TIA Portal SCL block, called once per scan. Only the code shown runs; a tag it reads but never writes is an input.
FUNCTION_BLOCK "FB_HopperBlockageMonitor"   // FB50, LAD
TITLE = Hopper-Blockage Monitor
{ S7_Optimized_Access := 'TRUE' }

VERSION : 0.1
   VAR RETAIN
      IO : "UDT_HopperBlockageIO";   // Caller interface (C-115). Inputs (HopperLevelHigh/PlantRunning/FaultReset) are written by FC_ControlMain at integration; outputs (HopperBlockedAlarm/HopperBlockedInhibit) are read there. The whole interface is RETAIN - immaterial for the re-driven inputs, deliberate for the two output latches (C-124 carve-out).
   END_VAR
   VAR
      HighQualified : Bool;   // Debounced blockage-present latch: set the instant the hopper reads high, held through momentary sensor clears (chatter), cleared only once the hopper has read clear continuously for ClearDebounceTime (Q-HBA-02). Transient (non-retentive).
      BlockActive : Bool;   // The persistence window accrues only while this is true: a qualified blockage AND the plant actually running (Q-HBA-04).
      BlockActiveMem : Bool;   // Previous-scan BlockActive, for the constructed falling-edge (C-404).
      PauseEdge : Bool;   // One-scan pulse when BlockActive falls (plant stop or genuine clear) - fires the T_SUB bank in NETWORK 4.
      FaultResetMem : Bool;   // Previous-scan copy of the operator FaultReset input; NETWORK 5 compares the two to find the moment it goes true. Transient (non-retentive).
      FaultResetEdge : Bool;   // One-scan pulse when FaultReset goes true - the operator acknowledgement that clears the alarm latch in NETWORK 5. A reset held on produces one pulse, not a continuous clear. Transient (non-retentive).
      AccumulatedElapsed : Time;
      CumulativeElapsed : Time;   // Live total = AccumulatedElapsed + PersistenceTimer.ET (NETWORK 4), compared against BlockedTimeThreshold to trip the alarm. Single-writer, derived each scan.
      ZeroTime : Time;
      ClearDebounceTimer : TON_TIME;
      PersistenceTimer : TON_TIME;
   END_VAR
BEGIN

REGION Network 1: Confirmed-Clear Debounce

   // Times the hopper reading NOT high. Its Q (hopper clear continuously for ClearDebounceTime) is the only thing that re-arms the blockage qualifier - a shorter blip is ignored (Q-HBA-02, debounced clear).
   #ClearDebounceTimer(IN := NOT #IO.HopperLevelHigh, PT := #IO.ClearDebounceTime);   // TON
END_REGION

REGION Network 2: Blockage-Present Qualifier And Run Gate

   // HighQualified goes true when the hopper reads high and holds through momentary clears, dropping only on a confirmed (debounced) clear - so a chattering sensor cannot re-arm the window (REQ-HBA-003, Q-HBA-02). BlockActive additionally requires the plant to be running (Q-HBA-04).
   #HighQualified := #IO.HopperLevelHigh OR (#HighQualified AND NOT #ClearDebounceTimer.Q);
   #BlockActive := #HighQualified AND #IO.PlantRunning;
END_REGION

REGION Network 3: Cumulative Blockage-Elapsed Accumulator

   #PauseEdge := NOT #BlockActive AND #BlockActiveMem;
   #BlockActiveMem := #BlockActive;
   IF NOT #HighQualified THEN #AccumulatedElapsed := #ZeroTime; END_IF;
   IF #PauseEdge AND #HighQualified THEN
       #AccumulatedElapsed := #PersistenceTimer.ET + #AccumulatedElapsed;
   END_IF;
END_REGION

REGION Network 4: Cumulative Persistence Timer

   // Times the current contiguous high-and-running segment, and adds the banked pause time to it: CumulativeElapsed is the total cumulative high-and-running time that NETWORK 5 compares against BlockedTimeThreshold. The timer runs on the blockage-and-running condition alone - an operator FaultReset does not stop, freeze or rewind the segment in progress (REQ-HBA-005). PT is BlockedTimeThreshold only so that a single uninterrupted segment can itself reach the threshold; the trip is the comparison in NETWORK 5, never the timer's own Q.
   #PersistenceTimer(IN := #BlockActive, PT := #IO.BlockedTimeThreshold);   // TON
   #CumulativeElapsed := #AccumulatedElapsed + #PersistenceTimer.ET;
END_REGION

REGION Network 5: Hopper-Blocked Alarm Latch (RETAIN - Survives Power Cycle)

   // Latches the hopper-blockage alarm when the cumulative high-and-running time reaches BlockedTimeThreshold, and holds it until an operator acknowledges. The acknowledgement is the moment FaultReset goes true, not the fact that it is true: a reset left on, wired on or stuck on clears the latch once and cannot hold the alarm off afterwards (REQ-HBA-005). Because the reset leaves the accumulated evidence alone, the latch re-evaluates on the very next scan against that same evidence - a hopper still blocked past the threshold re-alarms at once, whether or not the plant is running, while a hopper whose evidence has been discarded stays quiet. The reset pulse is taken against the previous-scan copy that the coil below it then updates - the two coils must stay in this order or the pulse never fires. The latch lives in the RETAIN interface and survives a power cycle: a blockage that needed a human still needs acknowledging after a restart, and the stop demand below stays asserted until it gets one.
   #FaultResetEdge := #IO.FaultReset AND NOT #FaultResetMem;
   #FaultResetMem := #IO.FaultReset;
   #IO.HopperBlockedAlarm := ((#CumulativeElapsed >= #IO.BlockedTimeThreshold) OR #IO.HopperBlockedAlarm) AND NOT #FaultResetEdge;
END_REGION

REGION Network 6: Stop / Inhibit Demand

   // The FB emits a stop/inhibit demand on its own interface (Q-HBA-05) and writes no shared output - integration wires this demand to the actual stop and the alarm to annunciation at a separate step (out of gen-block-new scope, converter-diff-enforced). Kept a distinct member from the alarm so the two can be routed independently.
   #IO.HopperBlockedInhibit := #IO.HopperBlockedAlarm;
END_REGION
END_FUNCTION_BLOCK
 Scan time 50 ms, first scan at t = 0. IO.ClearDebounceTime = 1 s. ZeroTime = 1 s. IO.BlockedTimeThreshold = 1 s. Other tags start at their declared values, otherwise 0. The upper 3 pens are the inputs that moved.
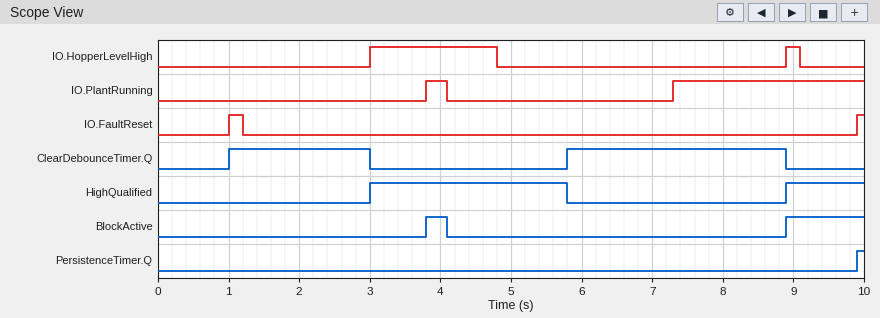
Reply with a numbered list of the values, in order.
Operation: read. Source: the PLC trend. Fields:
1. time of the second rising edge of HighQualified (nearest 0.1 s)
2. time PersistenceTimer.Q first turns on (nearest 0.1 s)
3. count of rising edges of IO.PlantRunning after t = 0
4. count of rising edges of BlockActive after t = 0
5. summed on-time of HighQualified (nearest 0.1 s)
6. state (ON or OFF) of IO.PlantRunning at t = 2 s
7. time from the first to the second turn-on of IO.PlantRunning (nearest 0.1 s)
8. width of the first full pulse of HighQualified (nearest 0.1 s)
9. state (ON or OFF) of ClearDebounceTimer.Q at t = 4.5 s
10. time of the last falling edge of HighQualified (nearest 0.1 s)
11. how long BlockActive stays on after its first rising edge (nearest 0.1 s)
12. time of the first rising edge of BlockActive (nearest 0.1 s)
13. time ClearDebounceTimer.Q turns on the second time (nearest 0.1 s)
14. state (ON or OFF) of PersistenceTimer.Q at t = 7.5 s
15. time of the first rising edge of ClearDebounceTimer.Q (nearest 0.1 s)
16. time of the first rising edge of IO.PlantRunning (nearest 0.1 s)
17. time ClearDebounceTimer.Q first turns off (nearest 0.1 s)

1. 8.9 s
2. 9.9 s
3. 2
4. 2
5. 3.9 s
6. OFF
7. 3.5 s
8. 2.8 s
9. OFF
10. 5.8 s
11. 0.3 s
12. 3.8 s
13. 5.8 s
14. OFF
15. 1.0 s
16. 3.8 s
17. 3.0 s
